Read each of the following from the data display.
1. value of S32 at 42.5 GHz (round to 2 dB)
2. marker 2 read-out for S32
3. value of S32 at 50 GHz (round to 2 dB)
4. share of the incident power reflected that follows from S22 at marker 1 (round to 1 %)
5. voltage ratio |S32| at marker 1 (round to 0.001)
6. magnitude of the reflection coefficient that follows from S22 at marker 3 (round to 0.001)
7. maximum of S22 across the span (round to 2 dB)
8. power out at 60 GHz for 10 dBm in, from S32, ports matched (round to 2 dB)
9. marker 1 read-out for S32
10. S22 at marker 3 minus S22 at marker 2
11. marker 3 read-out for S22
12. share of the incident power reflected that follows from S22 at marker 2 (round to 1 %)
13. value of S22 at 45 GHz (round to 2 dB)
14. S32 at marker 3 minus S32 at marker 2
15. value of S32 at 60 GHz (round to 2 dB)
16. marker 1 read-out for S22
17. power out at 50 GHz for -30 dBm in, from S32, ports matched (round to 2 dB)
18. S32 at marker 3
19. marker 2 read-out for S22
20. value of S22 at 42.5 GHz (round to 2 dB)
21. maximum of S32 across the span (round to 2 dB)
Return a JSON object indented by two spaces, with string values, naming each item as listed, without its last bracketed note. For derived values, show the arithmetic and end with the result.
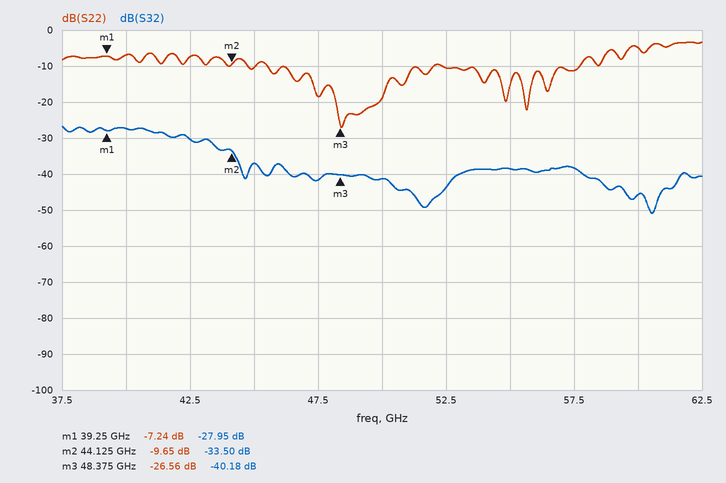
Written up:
{
  "value of S32 at 42.5 GHz": "-30 dB",
  "marker 2 read-out for S32": "-33.50 dB",
  "value of S32 at 50 GHz": "-42 dB",
  "share of the incident power reflected that follows from S22 at marker 1": "10^(-7.24/10) ≈ 19 %",
  "voltage ratio |S32| at marker 1": "10^(-27.95/20) ≈ 0.040",
  "magnitude of the reflection coefficient that follows from S22 at marker 3": "10^(-26.56/20) ≈ 0.047",
  "maximum of S22 across the span": "-4 dB",
  "power out at 60 GHz for 10 dBm in, from S32, ports matched": "10 dBm + (-46 dB) = -36 dBm",
  "marker 1 read-out for S32": "-27.95 dB",
  "S22 at marker 3 minus S22 at marker 2": "-26.56 − (-9.65) = -16.91 dB",
  "marker 3 read-out for S22": "-26.56 dB",
  "share of the incident power reflected that follows from S22 at marker 2": "10^(-9.65/10) ≈ 11 %",
  "value of S22 at 45 GHz": "-10 dB",
  "S32 at marker 3 minus S32 at marker 2": "-40.18 − (-33.5) = -6.68 dB",
  "value of S32 at 60 GHz": "-46 dB",
  "marker 1 read-out for S22": "-7.24 dB",
  "power out at 50 GHz for -30 dBm in, from S32, ports matched": "-30 dBm + (-42 dB) = -72 dBm",
  "S32 at marker 3": "-40.18 dB",
  "marker 2 read-out for S22": "-9.65 dB",
  "value of S22 at 42.5 GHz": "-8 dB",
  "maximum of S32 across the span": "-26 dB"
}
